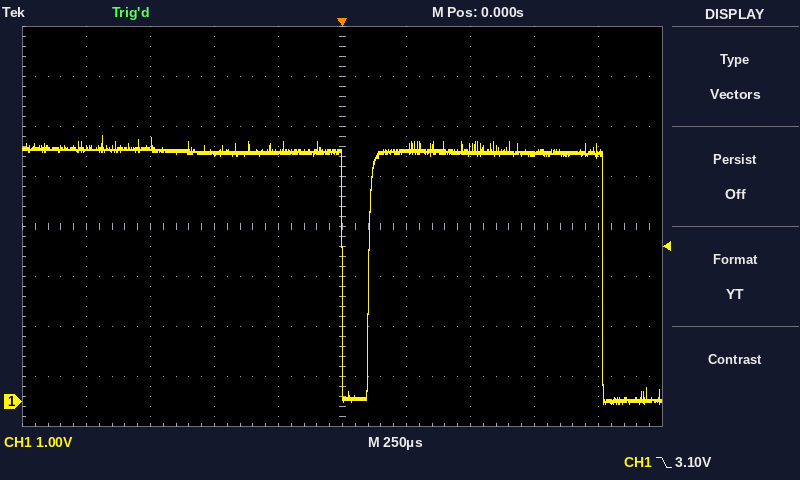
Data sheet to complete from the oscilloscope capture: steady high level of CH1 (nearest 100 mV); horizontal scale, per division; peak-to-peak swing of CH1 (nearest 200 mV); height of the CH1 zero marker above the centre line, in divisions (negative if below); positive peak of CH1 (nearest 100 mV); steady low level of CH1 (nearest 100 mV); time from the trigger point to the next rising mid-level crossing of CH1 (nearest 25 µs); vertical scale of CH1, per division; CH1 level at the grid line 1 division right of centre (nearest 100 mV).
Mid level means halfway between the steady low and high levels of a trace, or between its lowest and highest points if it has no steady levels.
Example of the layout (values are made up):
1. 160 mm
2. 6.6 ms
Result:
1. 5.0 V
2. 250 µs
3. 5.4 V
4. -3.5 div
5. 5.3 V
6. 0.0 V
7. 100 µs
8. 1 V
9. 5.0 V
